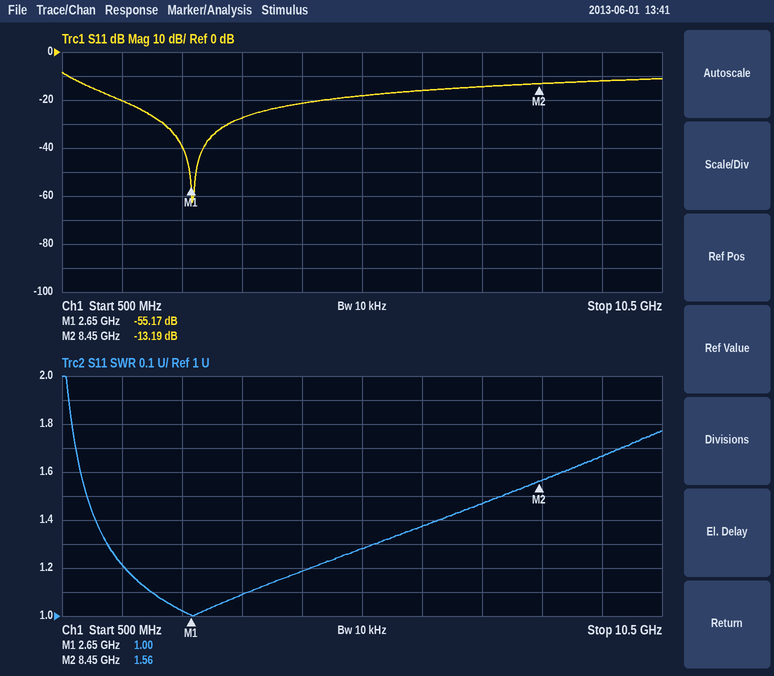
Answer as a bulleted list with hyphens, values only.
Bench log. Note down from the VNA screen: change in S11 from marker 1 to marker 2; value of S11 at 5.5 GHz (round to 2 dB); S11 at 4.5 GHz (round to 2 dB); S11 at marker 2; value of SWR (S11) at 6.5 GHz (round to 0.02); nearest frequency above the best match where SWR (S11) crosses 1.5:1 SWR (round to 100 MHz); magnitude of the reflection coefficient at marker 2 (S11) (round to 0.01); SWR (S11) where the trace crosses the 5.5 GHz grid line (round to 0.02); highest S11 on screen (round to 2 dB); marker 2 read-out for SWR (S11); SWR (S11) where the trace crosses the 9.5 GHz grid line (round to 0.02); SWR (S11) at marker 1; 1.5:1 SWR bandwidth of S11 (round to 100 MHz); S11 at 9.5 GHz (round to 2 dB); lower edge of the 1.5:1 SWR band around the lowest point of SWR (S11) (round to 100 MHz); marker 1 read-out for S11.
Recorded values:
- 41.98 dB
- -18 dB
- -22 dB
- -13.19 dB
- 1.38
- 7.8 GHz
- 0.22
- 1.28
- -8 dB
- 1.56
- 1.66
- 1.00
- 6.9 GHz
- -12 dB
- 900 MHz
- -55.17 dB
